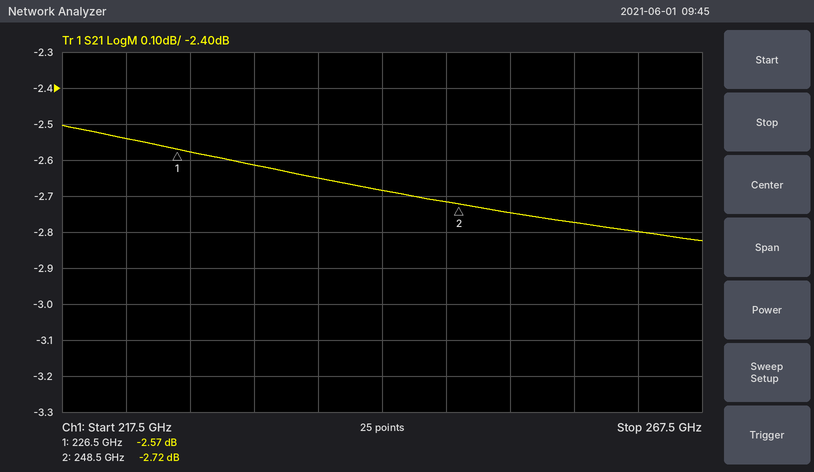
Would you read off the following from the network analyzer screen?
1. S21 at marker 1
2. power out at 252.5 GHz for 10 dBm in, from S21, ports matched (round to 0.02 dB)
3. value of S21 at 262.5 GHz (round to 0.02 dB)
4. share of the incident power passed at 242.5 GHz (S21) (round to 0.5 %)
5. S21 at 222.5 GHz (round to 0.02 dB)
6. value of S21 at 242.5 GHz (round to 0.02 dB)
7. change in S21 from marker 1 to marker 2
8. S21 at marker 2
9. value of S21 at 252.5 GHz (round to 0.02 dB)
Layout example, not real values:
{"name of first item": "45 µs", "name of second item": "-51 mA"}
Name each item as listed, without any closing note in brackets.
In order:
{"S21 at marker 1": "-2.57 dB", "power out at 252.5 GHz for 10 dBm in, from S21, ports matched": "7.26 dBm", "value of S21 at 262.5 GHz": "-2.80 dB", "share of the incident power passed at 242.5 GHz (S21)": "54.0 %", "S21 at 222.5 GHz": "-2.54 dB", "value of S21 at 242.5 GHz": "-2.68 dB", "change in S21 from marker 1 to marker 2": "-0.15 dB", "S21 at marker 2": "-2.72 dB", "value of S21 at 252.5 GHz": "-2.74 dB"}
